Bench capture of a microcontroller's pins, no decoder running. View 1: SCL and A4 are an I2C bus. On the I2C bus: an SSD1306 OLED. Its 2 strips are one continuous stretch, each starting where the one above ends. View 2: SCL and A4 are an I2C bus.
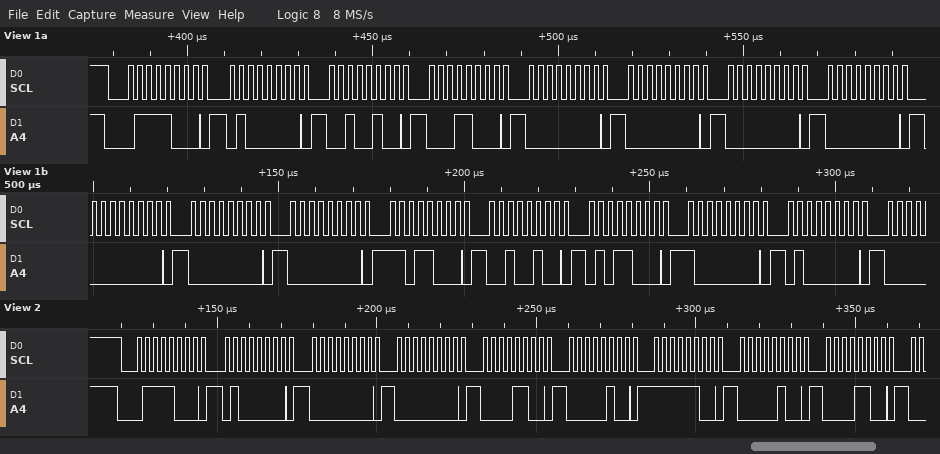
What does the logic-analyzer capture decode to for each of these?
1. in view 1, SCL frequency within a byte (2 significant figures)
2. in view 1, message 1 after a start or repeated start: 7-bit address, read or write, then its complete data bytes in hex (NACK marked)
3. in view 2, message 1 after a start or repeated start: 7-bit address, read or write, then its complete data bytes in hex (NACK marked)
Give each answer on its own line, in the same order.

400 kHz
0x3C write: 40 24 18 00 00 00 00 00 00 00 D8 24 58 80 40
0x3C write: 40 00 00 0C 04 FC 04 0C
